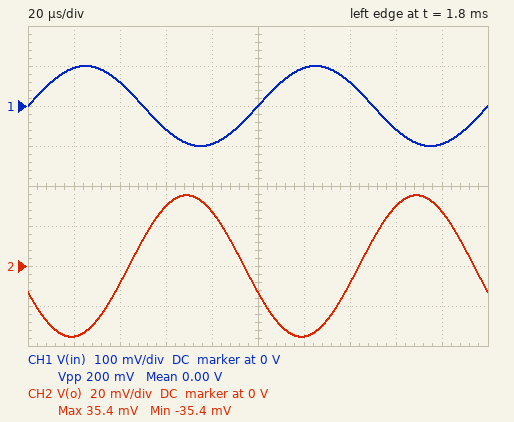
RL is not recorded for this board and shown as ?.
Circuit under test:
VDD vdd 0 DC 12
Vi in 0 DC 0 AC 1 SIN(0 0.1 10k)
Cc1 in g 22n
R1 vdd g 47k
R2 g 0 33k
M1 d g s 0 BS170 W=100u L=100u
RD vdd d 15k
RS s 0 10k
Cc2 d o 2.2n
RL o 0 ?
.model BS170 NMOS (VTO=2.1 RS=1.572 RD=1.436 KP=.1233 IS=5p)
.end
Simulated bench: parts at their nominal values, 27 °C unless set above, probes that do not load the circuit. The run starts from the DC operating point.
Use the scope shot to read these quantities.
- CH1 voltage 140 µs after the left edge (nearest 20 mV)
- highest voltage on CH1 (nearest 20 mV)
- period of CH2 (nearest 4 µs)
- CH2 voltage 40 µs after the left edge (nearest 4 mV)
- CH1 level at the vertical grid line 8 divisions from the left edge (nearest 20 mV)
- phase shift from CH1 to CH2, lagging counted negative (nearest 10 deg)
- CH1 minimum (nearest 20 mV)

60 mV
100 mV
100 µs
-8 mV
-60 mV
-160 deg
-100 mV
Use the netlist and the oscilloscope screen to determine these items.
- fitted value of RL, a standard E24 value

5.1 kΩ
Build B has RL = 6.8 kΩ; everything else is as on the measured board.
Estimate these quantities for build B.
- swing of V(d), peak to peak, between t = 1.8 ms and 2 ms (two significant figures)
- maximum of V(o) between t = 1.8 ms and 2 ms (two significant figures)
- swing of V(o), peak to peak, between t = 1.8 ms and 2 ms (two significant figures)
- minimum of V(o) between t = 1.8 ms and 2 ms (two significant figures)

130 mV
44 mV
88 mV
-44 mV
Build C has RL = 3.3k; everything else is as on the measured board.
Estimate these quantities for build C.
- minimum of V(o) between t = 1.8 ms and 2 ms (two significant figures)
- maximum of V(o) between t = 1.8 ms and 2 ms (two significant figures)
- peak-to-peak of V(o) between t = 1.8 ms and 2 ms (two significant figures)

-25 mV
25 mV
50 mV
